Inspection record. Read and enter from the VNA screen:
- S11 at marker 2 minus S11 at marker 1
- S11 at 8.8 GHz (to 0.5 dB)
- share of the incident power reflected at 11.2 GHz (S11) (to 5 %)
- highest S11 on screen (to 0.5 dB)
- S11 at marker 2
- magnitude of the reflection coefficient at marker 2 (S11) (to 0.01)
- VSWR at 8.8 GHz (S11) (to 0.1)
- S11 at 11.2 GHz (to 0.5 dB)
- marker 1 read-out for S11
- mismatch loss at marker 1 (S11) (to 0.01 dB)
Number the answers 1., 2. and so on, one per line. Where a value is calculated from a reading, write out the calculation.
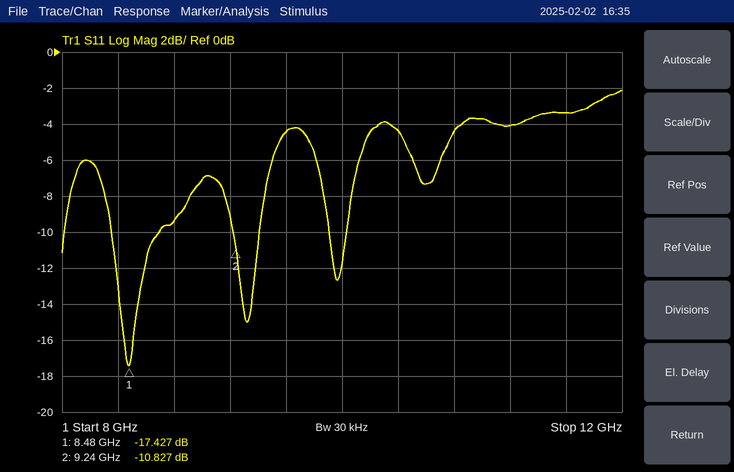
1. -10.827 − (-17.427) = 6.600 dB
2. -9.5 dB
3. 10^(-4/10) ≈ 40 %
4. -2.0 dB
5. -10.827 dB
6. 10^(-10.827/20) ≈ 0.29
7. |Γ| = 10^(-9.5/20) = 0.3350; VSWR = (1 + 0.3350)/(1 − 0.3350) ≈ 2.0
8. -4.0 dB
9. -17.427 dB
10. −10 log10(1 − 10^(-17.427/10)) ≈ 0.08 dB
